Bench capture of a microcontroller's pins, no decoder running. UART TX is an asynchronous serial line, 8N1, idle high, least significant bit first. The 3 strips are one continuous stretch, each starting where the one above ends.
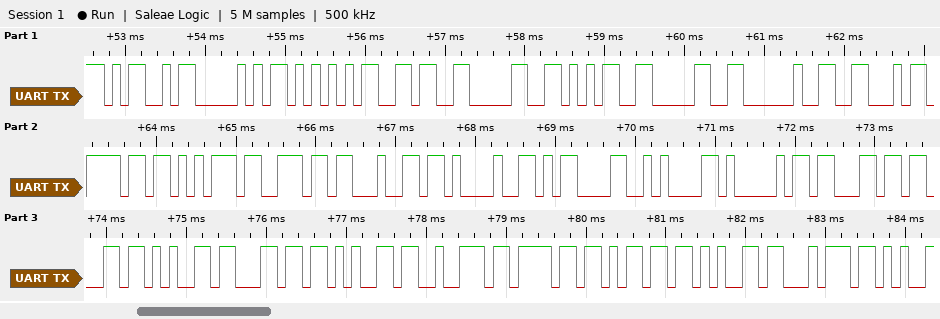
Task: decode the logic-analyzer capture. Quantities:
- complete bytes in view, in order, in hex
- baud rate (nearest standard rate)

4D 50 55 36 30 35 30 20 46 6F 75 6E 64 21 0D 0A 41 63 63 65 6C 65 72 6F 6D 65 74
9600 baud
